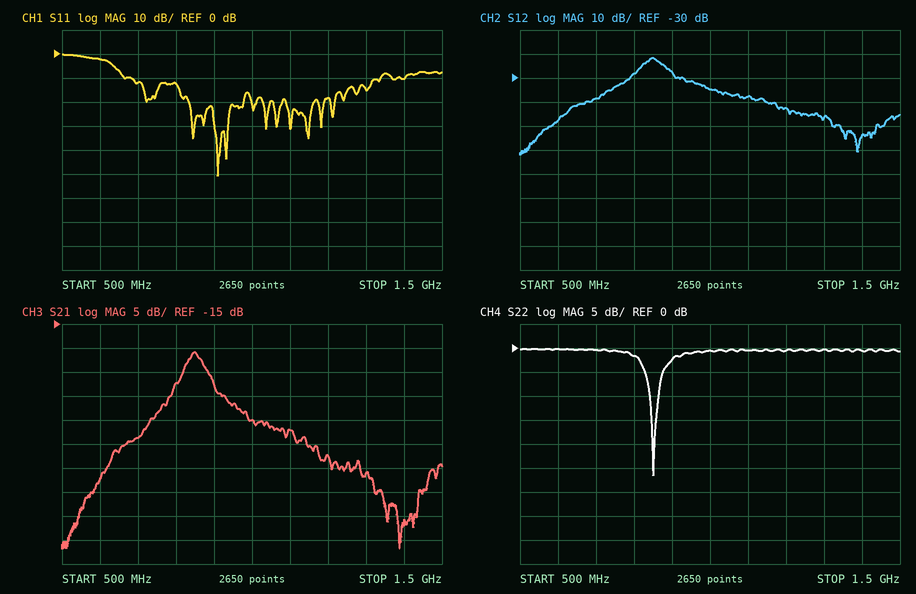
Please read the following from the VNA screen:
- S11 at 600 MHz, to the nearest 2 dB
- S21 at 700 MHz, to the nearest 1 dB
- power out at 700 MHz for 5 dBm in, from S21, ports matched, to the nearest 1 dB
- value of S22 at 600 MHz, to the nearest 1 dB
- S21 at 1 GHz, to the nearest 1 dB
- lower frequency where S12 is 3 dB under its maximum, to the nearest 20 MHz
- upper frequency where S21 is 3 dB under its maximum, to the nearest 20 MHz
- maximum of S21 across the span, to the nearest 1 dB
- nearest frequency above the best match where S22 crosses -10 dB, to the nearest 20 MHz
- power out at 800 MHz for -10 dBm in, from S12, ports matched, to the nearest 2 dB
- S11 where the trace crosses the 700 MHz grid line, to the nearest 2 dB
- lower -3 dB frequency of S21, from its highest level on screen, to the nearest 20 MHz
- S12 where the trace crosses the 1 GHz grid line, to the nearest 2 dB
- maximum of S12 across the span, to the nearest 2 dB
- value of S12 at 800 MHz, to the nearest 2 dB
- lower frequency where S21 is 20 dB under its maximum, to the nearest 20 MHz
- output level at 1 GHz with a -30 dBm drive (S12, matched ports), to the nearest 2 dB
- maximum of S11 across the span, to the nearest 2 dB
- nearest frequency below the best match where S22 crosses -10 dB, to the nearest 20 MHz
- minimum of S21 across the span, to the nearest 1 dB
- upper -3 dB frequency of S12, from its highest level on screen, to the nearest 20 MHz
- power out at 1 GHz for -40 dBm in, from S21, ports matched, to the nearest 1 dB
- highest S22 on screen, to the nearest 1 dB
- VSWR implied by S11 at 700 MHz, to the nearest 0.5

-2 dB
-39 dB
-34 dBm
0 dB
-35 dB
820 MHz
880 MHz
-21 dB
860 MHz
-38 dBm
-12 dB
820 MHz
-34 dB
-22 dB
-28 dB
660 MHz
-64 dBm
0 dB
840 MHz
-62 dB
880 MHz
-75 dBm
0 dB
1.5
